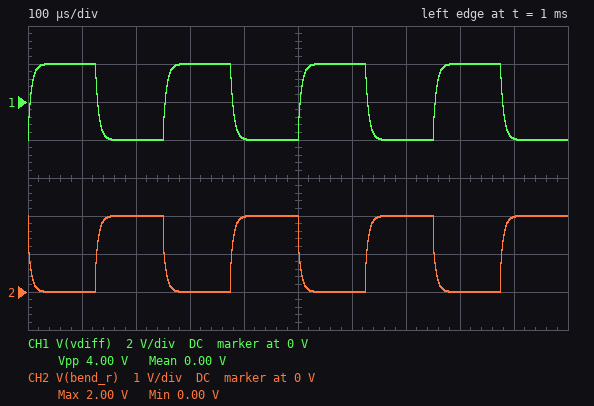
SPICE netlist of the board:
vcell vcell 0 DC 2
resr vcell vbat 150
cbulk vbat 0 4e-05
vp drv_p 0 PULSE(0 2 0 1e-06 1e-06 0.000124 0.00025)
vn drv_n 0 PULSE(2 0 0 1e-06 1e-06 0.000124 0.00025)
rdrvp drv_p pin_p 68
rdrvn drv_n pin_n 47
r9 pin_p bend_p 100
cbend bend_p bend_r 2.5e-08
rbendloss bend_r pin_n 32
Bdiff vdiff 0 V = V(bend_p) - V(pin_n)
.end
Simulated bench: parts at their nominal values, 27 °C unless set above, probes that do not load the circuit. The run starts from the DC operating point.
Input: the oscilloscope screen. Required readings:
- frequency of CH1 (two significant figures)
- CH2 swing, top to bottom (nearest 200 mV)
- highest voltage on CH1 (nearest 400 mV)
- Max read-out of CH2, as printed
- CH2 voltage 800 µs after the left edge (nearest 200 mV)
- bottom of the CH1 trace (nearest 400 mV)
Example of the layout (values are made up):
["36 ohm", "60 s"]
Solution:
["4.0 kHz", "2.0 V", "2.0 V", "2.00 V", "0 V", "-2.0 V"]
